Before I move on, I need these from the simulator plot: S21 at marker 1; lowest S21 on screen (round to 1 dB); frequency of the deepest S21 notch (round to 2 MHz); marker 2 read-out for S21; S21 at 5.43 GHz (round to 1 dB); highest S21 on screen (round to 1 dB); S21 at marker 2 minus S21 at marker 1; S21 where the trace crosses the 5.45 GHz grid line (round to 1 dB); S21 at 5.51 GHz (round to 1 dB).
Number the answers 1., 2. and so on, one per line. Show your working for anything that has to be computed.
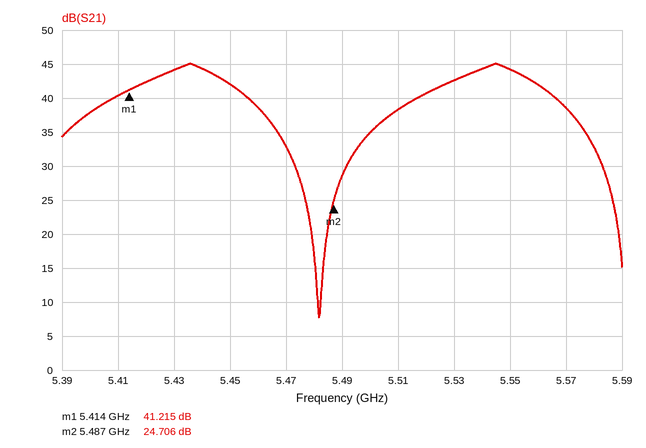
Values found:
1. 41.215 dB
2. 8 dB
3. 5.482 GHz
4. 24.706 dB
5. 44 dB
6. 45 dB
7. 24.706 − (41.215) = -16.509 dB
8. 42 dB
9. 38 dB
